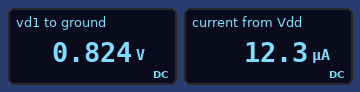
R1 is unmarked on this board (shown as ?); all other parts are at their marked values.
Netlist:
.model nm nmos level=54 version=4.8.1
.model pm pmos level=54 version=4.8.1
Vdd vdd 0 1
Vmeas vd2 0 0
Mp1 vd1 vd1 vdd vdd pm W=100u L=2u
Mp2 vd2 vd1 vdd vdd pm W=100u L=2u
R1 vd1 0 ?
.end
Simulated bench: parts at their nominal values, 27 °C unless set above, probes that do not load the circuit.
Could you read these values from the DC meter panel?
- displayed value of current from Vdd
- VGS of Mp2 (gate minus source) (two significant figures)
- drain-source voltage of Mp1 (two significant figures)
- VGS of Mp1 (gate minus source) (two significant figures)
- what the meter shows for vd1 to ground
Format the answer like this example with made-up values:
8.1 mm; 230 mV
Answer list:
12.3 µA; -180 mV; -180 mV; -180 mV; 0.824 V
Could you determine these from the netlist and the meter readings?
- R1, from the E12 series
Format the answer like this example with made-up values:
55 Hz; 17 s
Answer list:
150 kΩ
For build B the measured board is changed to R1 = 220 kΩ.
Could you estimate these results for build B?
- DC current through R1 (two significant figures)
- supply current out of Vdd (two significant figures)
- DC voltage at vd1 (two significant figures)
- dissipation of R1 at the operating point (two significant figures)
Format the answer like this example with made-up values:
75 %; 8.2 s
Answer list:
3.8 µA; 8.6 µA; 840 mV; 3.2 µW
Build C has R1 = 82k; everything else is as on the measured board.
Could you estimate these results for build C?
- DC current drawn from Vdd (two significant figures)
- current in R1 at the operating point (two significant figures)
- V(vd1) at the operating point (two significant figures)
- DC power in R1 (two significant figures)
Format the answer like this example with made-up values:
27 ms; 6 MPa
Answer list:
22 µA; 9.8 µA; 800 mV; 7.9 µW
